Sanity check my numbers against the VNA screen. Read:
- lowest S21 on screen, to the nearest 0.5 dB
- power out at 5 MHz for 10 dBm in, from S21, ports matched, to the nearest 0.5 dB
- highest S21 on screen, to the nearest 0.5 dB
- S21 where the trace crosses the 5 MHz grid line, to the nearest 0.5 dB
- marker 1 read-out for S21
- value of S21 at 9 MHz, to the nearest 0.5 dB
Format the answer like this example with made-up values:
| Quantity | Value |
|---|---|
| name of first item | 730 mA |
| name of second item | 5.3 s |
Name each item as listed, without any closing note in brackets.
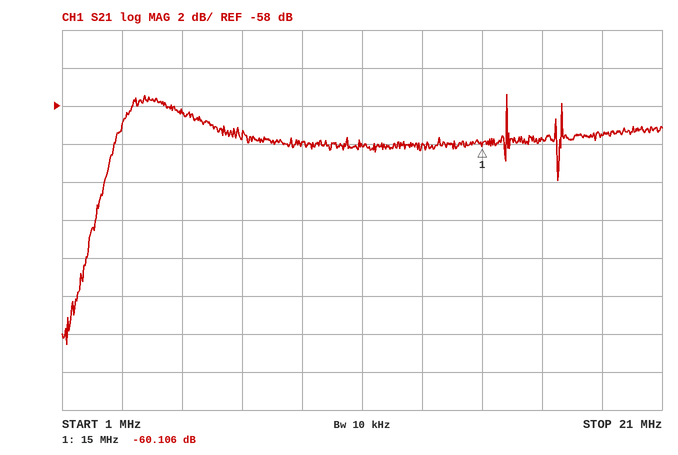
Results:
| Quantity | Value |
|---|---|
| lowest S21 on screen, to the nearest 0.5 dB | -70.5 dB |
| power out at 5 MHz for 10 dBm in, from S21, ports matched, to the nearest 0.5 dB | -48.5 dBm |
| highest S21 on screen, to the nearest 0.5 dB | -57.5 dB |
| S21 where the trace crosses the 5 MHz grid line, to the nearest 0.5 dB | -58.5 dB |
| marker 1 read-out for S21 | -60.106 dB |
| value of S21 at 9 MHz, to the nearest 0.5 dB | -60.0 dB |
